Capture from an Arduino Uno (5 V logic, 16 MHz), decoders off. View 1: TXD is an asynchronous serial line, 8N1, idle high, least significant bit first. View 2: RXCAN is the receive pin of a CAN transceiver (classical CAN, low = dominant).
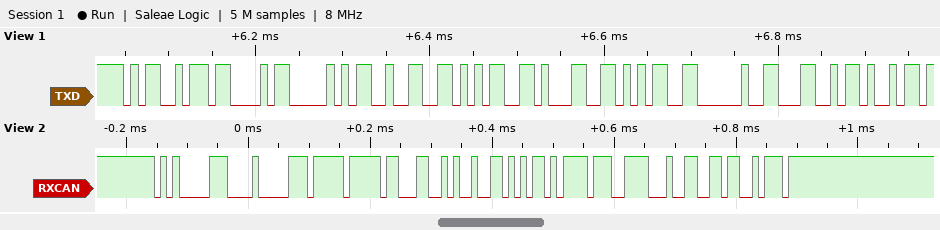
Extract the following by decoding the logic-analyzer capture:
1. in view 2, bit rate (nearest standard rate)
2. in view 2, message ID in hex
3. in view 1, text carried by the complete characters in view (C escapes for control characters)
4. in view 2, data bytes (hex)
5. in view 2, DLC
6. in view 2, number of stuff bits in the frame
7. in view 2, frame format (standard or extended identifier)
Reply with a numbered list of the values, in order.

1. 100 kbit/s
2. 0x506
3. "MCP2515 Li"
4. 37 FF 8C A4 D5 AF 73 C4
5. 8
6. 4
7. standard
